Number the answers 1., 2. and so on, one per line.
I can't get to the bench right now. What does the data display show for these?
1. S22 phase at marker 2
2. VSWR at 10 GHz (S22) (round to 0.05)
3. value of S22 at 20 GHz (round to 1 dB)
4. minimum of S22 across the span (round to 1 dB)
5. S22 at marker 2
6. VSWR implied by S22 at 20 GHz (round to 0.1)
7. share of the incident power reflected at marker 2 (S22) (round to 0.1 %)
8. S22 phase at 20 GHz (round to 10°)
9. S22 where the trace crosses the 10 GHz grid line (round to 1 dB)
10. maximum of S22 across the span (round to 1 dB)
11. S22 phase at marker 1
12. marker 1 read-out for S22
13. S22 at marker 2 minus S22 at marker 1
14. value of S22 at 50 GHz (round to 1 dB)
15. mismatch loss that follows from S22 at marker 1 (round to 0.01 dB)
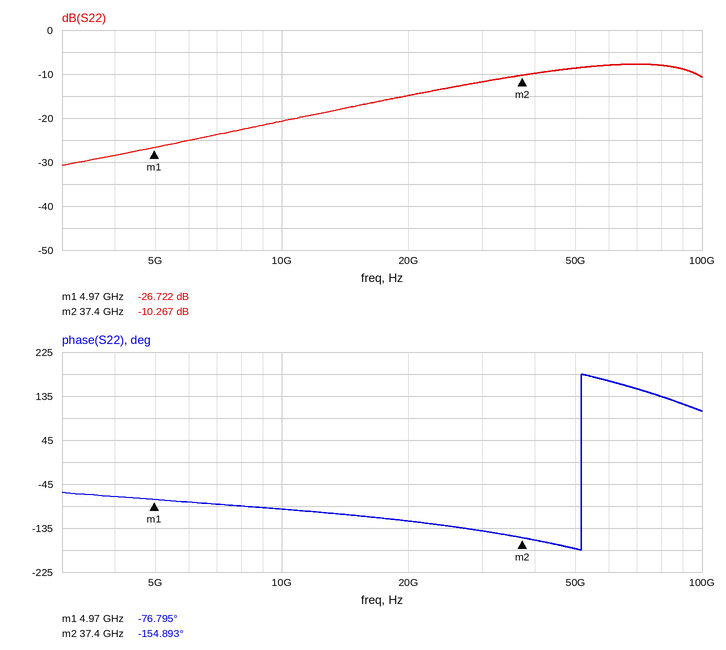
1. -154.893°
2. 1.20
3. -15 dB
4. -31 dB
5. -10.267 dB
6. 1.4
7. 9.4 %
8. -120°
9. -21 dB
10. -8 dB
11. -76.795°
12. -26.722 dB
13. 16.455 dB
14. -9 dB
15. 0.01 dB
